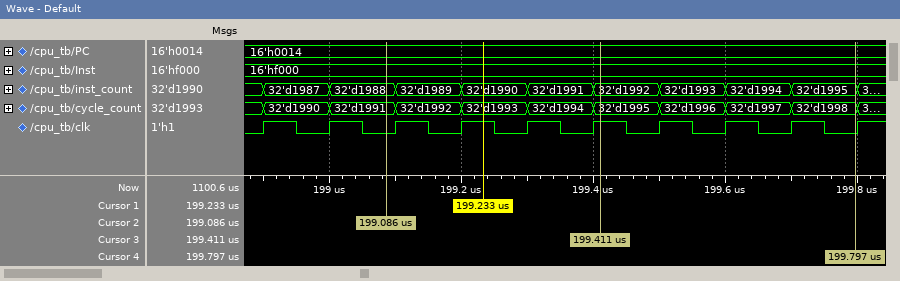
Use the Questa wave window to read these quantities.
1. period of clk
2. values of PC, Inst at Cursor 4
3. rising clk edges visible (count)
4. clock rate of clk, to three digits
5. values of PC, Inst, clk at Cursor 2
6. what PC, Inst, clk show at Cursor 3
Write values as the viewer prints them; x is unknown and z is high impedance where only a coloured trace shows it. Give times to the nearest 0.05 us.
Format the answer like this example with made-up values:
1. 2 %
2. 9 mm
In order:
1. 0.1 us
2. PC=16'h0014, Inst=16'hf000
3. 10
4. 10.0 MHz
5. PC=16'h0014, Inst=16'hf000, clk=0
6. PC=16'h0014, Inst=16'hf000, clk=1
